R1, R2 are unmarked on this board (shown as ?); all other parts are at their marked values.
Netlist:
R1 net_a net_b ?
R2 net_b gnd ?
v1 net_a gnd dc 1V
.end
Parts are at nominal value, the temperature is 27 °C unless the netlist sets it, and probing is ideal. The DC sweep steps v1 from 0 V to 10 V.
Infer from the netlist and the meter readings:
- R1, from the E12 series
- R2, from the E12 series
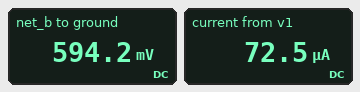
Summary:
5.6 kΩ
8.2 kΩ
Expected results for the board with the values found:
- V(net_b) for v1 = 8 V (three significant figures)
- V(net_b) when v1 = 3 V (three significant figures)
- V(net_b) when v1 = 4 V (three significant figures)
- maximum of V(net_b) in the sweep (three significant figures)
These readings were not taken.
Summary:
4.75 V
1.78 V
2.38 V
5.94 V
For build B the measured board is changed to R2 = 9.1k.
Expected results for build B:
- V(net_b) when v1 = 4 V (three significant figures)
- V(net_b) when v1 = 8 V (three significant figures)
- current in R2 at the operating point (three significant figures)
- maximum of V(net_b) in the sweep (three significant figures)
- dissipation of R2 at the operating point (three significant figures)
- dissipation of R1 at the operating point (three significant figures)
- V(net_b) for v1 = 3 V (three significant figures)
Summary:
2.48 V
4.95 V
68.0 µA
6.19 V
42.1 µW
25.9 µW
1.86 V
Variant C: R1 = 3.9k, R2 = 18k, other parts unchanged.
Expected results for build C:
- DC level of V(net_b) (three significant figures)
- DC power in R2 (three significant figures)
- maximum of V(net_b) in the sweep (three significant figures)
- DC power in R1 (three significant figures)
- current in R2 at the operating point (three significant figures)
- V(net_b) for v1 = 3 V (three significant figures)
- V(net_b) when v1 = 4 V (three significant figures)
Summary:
822 mV
37.5 µW
8.22 V
8.13 µW
45.7 µA
2.47 V
3.29 V
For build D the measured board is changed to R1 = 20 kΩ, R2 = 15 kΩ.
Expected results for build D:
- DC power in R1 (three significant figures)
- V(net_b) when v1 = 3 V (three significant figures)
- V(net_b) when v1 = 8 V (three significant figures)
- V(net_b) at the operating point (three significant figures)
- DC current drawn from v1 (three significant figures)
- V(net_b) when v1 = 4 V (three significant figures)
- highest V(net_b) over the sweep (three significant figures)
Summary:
16.3 µW
1.29 V
3.43 V
429 mV
28.6 µA
1.71 V
4.29 V
